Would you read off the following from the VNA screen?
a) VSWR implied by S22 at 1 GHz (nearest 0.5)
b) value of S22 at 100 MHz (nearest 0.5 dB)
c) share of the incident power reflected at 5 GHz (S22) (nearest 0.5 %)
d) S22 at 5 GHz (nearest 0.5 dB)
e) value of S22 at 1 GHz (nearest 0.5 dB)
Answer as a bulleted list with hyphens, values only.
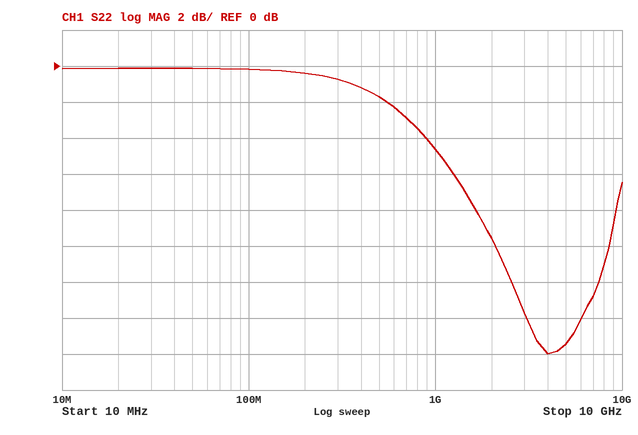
- 4.0
- 0.0 dB
- 3.0 %
- -15.5 dB
- -4.5 dB
